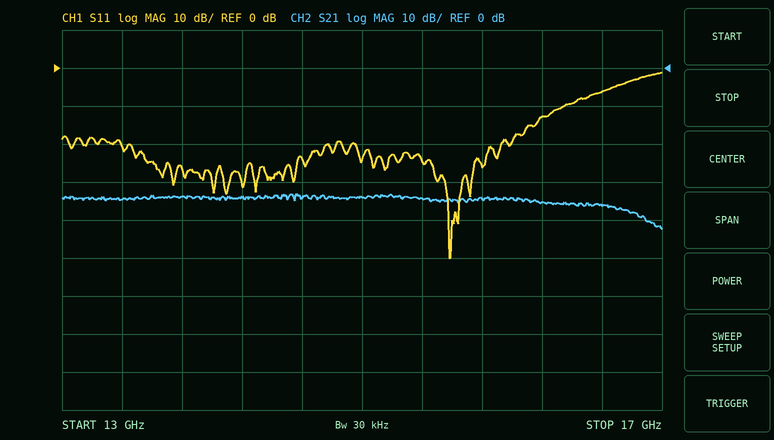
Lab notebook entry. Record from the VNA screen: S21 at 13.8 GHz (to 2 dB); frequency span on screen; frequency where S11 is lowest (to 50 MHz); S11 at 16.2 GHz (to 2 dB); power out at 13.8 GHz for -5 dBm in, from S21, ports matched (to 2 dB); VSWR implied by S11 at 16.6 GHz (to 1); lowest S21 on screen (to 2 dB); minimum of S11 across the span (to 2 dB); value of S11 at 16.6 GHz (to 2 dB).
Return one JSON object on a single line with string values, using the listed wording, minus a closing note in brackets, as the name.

{"S21 at 13.8 GHz": "-34 dB", "frequency span on screen": "4 GHz", "frequency where S11 is lowest": "15.60 GHz", "S11 at 16.2 GHz": "-12 dB", "power out at 13.8 GHz for -5 dBm in, from S21, ports matched": "-38 dBm", "VSWR implied by S11 at 16.6 GHz": "3", "lowest S21 on screen": "-42 dB", "minimum of S11 across the span": "-50 dB", "value of S11 at 16.6 GHz": "-6 dB"}
